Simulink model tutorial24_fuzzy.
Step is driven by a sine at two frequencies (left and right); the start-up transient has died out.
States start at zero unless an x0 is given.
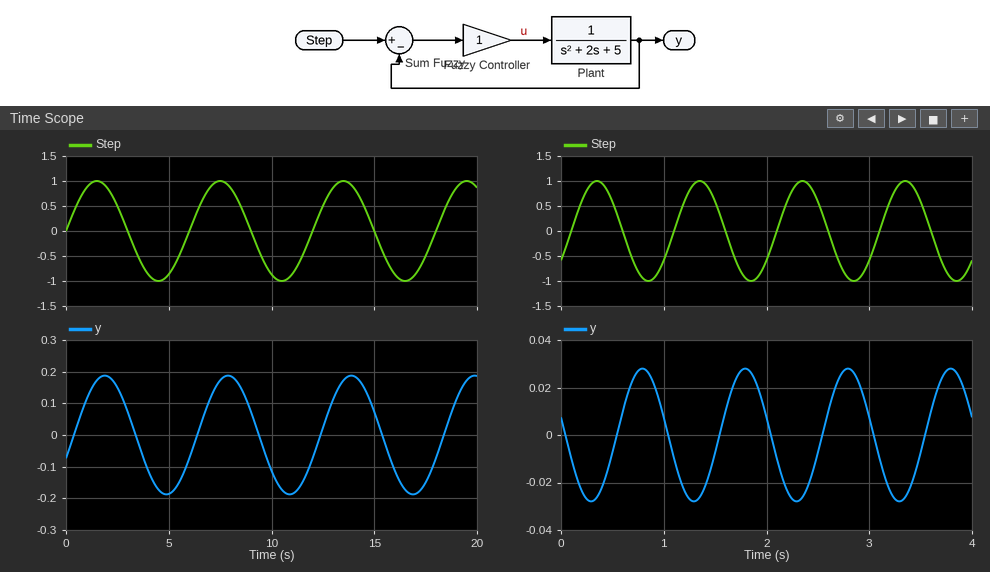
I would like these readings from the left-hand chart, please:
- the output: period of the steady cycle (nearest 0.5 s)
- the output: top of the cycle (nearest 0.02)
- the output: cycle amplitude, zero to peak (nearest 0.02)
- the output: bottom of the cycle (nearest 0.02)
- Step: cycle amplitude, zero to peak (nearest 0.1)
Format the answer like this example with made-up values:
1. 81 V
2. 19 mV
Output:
1. 6.0 s
2. 0.18
3. 0.18
4. -0.18
5. 1.0
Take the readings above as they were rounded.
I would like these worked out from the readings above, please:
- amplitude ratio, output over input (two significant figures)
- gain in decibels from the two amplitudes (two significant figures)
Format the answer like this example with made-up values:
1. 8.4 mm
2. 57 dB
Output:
1. 0.18
2. -15 dB
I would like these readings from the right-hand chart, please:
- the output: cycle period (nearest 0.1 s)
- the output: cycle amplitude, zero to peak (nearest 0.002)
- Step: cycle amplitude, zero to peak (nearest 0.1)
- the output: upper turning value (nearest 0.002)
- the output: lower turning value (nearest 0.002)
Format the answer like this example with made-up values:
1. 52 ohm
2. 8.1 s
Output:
1. 1.0 s
2. 0.028
3. 1.0
4. 0.028
5. -0.028
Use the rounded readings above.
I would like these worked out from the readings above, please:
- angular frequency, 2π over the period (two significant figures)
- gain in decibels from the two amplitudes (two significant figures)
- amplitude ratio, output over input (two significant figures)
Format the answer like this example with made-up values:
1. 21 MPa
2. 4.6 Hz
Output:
1. 6.3 rad/s
2. -31 dB
3. 0.028
